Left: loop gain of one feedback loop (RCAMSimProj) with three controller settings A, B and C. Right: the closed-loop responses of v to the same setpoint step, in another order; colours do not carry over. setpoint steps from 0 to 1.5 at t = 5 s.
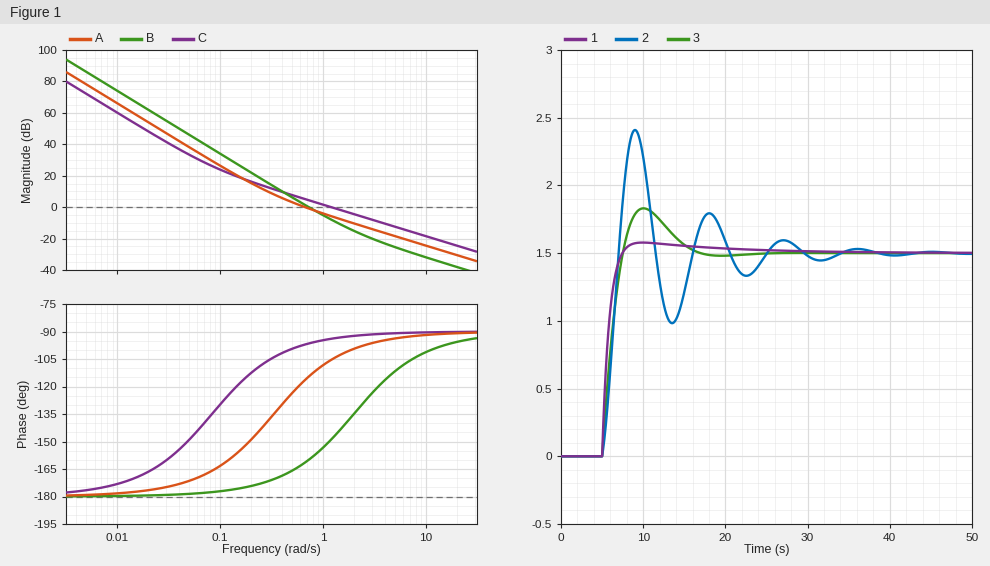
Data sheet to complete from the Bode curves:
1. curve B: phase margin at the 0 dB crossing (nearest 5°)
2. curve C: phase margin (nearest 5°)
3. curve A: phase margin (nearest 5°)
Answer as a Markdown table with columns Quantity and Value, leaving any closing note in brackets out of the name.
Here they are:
| Quantity | Value |
|---|---|
| curve B: phase margin at the 0 dB crossing | 20° |
| curve C: phase margin | 85° |
| curve A: phase margin | 65° |
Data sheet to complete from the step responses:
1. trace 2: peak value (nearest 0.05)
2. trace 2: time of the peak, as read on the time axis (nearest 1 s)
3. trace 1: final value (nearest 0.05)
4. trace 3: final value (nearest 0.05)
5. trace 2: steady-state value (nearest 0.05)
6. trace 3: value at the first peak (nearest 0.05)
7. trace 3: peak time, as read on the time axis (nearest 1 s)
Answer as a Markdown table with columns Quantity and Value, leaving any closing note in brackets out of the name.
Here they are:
| Quantity | Value |
|---|---|
| trace 2: peak value | 2.40 |
| trace 2: time of the peak, as read on the time axis | 9 s |
| trace 1: final value | 1.50 |
| trace 3: final value | 1.50 |
| trace 2: steady-state value | 1.50 |
| trace 3: value at the first peak | 1.85 |
| trace 3: peak time, as read on the time axis | 10 s |
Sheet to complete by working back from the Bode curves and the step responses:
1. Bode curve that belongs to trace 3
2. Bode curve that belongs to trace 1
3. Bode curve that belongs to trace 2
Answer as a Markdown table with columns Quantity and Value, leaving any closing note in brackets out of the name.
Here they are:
| Quantity | Value |
|---|---|
| Bode curve that belongs to trace 3 | A |
| Bode curve that belongs to trace 1 | C |
| Bode curve that belongs to trace 2 | B |
